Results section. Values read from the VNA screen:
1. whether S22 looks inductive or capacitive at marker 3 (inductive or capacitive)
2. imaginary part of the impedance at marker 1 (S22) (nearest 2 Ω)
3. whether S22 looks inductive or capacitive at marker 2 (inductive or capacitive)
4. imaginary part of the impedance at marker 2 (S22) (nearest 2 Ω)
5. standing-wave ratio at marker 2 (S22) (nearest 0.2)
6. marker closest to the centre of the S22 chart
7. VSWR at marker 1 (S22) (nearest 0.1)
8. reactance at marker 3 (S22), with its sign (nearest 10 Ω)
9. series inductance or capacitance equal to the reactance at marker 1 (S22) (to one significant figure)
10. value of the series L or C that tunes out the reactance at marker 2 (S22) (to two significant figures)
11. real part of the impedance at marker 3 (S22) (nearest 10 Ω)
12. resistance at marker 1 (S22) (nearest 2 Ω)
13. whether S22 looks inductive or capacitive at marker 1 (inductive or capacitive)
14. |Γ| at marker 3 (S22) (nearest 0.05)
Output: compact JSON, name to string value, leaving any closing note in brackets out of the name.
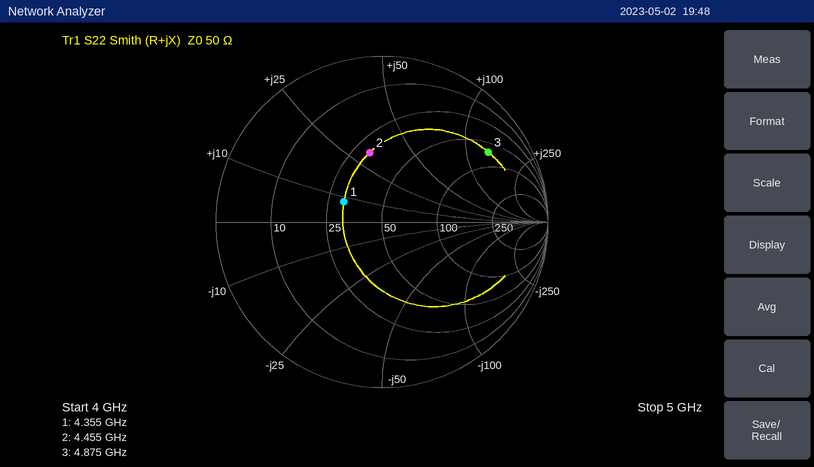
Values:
{"whether S22 looks inductive or capacitive at marker 3": "inductive", "imaginary part of the impedance at marker 1 (S22)": "+8 Ω", "whether S22 looks inductive or capacitive at marker 2": "inductive", "imaginary part of the impedance at marker 2 (S22)": "+32 Ω", "standing-wave ratio at marker 2 (S22)": "2.4", "marker closest to the centre of the S22 chart": "marker 1", "VSWR at marker 1 (S22)": "1.7", "reactance at marker 3 (S22), with its sign": "+140 Ω", "series inductance or capacitance equal to the reactance at marker 1 (S22)": "300 pH", "value of the series L or C that tunes out the reactance at marker 2 (S22)": "1.1 pF", "real part of the impedance at marker 3 (S22)": "70 Ω", "resistance at marker 1 (S22)": "30 Ω", "whether S22 looks inductive or capacitive at marker 1": "inductive", "|Γ| at marker 3 (S22)": "0.75"}
